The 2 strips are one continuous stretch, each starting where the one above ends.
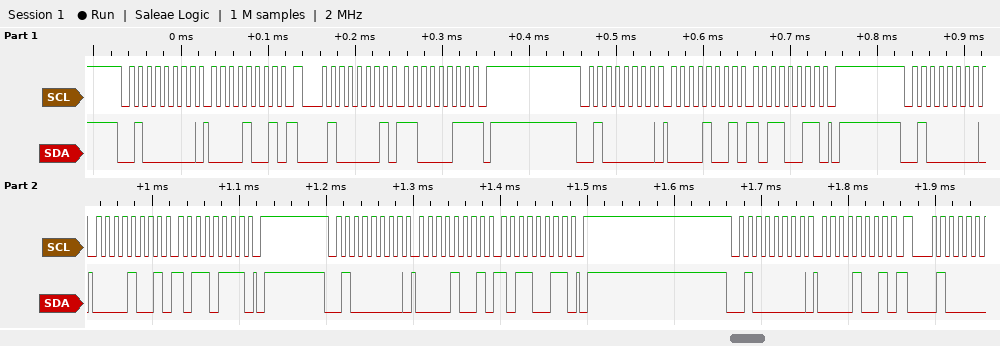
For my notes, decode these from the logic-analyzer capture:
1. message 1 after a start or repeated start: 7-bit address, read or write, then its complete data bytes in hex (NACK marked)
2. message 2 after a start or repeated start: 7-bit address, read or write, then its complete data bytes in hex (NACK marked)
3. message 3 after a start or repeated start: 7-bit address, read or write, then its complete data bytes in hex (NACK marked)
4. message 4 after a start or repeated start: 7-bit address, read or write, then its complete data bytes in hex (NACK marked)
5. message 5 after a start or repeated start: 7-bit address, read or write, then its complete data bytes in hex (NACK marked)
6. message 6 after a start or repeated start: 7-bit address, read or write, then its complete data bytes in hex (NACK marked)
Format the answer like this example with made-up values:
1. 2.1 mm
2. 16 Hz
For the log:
1. 0x20 write: 09
2. 0x20 read: C3 NACK
3. 0x20 write: 09 B3
4. 0x20 write: 09 B7
5. 0x20 write: 09 B3
6. 0x20 write: 09
